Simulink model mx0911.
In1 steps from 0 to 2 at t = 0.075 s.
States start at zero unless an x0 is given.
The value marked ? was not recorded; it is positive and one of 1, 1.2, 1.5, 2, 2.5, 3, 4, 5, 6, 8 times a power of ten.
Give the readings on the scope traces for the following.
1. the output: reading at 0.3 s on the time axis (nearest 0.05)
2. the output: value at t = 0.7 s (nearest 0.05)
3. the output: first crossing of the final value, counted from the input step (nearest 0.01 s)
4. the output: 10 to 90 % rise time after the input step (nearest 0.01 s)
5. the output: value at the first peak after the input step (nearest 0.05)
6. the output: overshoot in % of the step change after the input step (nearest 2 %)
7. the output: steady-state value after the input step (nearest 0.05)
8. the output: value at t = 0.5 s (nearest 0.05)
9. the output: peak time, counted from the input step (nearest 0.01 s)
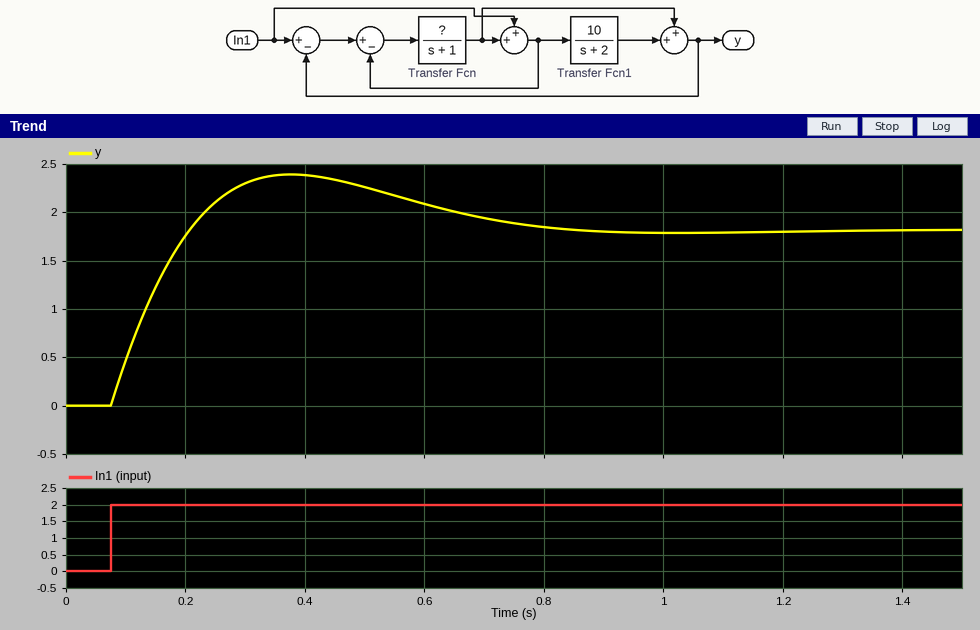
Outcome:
2.30
1.95
0.13 s
0.10 s
2.40
32 %
1.80
2.25
0.30 s
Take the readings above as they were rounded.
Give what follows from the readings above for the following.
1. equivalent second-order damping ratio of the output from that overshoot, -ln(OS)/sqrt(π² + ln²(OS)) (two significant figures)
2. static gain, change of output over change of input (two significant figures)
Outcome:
0.34
0.90
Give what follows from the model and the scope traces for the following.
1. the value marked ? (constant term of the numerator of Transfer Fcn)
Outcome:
3
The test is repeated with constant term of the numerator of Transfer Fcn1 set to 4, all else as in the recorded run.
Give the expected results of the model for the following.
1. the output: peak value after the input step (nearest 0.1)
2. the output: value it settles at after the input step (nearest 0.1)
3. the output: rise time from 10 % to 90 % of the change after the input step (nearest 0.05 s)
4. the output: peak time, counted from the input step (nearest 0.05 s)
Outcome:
1.3
1.2
0.25 s
0.55 s
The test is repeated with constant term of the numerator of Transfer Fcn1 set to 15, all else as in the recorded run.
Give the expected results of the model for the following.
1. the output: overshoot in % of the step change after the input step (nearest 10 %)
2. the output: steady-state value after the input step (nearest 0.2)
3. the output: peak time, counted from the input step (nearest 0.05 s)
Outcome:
50 %
2.0
0.25 s
